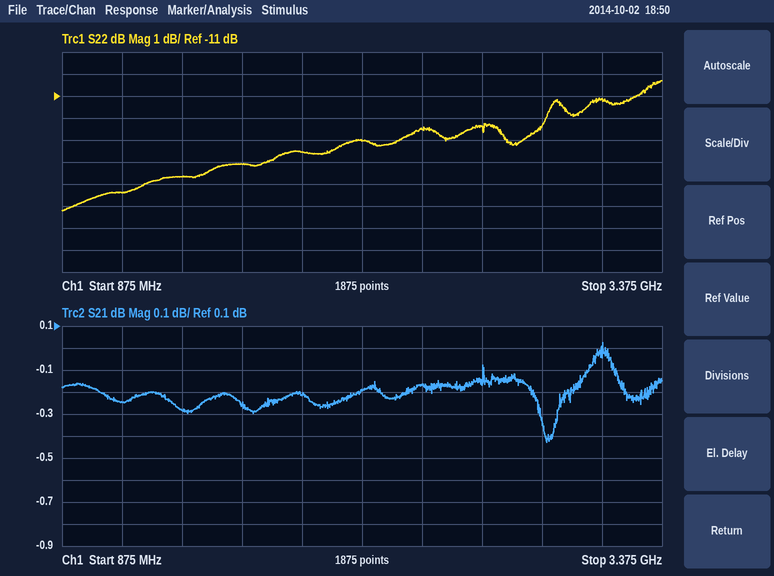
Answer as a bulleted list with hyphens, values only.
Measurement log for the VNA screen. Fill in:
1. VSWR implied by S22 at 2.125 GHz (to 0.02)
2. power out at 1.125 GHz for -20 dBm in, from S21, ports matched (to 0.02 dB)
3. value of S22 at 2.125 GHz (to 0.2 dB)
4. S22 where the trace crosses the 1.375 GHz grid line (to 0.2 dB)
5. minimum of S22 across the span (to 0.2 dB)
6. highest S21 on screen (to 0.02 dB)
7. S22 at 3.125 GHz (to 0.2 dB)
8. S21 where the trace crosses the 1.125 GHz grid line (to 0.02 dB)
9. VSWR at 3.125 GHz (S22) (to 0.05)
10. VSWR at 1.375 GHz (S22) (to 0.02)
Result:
- 1.58
- -20.24 dBm
- -13.0 dB
- -14.6 dB
- -16.2 dB
- 0.02 dB
- -11.2 dB
- -0.24 dB
- 1.75
- 1.46
